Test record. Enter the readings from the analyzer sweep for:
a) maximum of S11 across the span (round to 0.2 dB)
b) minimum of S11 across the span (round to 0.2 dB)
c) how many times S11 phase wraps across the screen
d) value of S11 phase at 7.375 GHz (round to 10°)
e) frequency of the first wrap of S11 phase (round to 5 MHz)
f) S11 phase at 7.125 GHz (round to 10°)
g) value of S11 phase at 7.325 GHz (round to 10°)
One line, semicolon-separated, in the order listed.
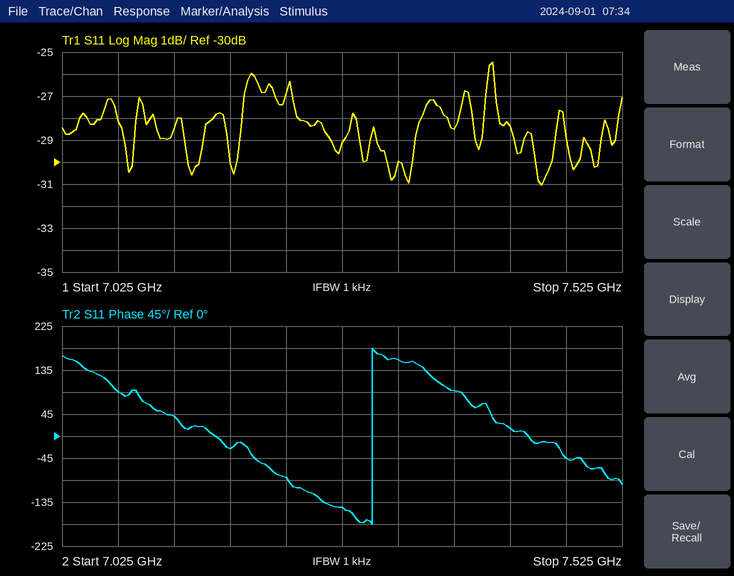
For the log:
-25.4 dB; -31.0 dB; 1; 90°; 7.300 GHz; 40°; 160°
